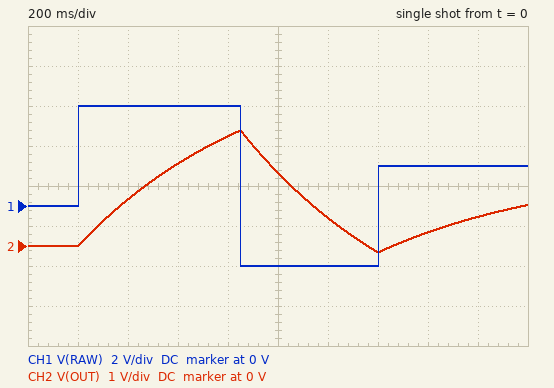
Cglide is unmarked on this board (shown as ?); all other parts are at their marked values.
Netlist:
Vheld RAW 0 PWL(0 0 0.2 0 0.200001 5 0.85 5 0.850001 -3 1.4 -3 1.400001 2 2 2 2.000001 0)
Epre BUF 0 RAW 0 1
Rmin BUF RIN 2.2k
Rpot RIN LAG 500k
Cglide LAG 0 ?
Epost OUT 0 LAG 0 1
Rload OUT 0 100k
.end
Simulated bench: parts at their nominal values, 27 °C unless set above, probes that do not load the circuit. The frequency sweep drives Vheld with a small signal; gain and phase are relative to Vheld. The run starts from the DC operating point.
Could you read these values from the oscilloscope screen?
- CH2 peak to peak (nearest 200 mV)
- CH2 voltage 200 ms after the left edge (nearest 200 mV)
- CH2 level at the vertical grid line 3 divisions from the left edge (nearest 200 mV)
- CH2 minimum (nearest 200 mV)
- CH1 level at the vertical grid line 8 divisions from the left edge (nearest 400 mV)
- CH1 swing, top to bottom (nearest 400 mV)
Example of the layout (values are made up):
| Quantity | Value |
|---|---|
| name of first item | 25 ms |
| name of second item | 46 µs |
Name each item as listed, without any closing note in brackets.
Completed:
| Quantity | Value |
|---|---|
| CH2 peak to peak | 3.0 V |
| CH2 voltage 200 ms after the left edge | 0 V |
| CH2 level at the vertical grid line 3 divisions from the left edge | 2.0 V |
| CH2 minimum | -200 mV |
| CH1 level at the vertical grid line 8 divisions from the left edge | 2.0 V |
| CH1 swing, top to bottom | 8.0 V |
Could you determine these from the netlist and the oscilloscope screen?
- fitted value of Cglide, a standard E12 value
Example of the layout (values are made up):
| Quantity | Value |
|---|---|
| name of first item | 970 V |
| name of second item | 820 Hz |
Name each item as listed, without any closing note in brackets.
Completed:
| Quantity | Value |
|---|---|
| fitted value of Cglide, a standard E12 value | 1.5 µF |
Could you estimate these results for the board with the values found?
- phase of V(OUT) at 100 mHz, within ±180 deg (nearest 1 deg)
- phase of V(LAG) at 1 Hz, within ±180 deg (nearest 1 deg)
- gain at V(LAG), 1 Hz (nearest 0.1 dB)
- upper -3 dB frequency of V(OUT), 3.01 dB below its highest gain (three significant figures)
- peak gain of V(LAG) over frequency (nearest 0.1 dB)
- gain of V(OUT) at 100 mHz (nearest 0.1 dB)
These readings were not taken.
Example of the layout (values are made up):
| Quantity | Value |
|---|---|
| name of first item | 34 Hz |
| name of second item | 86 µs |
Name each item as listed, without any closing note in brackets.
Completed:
| Quantity | Value |
|---|---|
| phase of V(OUT) at 100 mHz, within ±180 deg | -25 deg |
| phase of V(LAG) at 1 Hz, within ±180 deg | -78 deg |
| gain at V(LAG), 1 Hz | -13.7 dB |
| upper -3 dB frequency of V(OUT), 3.01 dB below its highest gain | 211 mHz |
| peak gain of V(LAG) over frequency | 0 dB |
| gain of V(OUT) at 100 mHz | -0.9 dB |
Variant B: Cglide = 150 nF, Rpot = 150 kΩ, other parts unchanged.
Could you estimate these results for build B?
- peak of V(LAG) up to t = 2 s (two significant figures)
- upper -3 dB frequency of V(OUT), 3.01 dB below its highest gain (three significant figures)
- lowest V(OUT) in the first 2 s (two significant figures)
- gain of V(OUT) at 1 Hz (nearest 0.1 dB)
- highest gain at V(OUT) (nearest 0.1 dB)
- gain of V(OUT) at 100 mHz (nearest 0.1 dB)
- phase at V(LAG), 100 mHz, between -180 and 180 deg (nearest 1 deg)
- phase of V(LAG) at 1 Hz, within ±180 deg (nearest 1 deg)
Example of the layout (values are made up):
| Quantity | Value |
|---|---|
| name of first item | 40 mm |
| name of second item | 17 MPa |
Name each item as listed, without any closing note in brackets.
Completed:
| Quantity | Value |
|---|---|
| peak of V(LAG) up to t = 2 s | 5.0 V |
| upper -3 dB frequency of V(OUT), 3.01 dB below its highest gain | 6.97 Hz |
| lowest V(OUT) in the first 2 s | -3.0 V |
| gain of V(OUT) at 1 Hz | -0.1 dB |
| highest gain at V(OUT) | 0 dB |
| gain of V(OUT) at 100 mHz | 0 dB |
| phase at V(LAG), 100 mHz, between -180 and 180 deg | -1 deg |
| phase of V(LAG) at 1 Hz, within ±180 deg | -8 deg |
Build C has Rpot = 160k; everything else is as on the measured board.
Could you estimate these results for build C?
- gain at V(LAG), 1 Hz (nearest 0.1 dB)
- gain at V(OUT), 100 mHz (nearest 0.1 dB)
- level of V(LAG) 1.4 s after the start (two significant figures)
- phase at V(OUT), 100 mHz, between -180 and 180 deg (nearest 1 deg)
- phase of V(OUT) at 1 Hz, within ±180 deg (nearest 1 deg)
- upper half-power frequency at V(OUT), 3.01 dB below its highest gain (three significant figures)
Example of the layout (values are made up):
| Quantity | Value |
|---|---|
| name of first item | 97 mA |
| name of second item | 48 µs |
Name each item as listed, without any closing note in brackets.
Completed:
| Quantity | Value |
|---|---|
| gain at V(LAG), 1 Hz | -5.2 dB |
| gain at V(OUT), 100 mHz | -0.1 dB |
| level of V(LAG) 1.4 s after the start | -2.2 V |
| phase at V(OUT), 100 mHz, between -180 and 180 deg | -9 deg |
| phase of V(OUT) at 1 Hz, within ±180 deg | -57 deg |
| upper half-power frequency at V(OUT), 3.01 dB below its highest gain | 654 mHz |
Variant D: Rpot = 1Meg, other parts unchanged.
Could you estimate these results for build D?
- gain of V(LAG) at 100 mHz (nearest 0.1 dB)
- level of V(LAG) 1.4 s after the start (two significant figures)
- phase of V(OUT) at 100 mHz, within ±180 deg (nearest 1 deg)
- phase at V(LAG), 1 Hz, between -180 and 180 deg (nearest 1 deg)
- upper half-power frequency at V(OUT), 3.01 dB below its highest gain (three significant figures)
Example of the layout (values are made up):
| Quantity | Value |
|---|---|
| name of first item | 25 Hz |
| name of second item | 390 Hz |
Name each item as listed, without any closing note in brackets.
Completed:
| Quantity | Value |
|---|---|
| gain of V(LAG) at 100 mHz | -2.8 dB |
| level of V(LAG) 1.4 s after the start | 300 mV |
| phase of V(OUT) at 100 mHz, within ±180 deg | -43 deg |
| phase at V(LAG), 1 Hz, between -180 and 180 deg | -84 deg |
| upper half-power frequency at V(OUT), 3.01 dB below its highest gain | 106 mHz |
